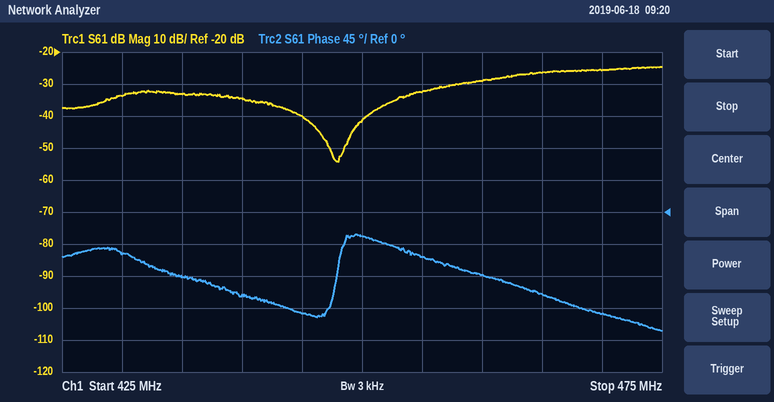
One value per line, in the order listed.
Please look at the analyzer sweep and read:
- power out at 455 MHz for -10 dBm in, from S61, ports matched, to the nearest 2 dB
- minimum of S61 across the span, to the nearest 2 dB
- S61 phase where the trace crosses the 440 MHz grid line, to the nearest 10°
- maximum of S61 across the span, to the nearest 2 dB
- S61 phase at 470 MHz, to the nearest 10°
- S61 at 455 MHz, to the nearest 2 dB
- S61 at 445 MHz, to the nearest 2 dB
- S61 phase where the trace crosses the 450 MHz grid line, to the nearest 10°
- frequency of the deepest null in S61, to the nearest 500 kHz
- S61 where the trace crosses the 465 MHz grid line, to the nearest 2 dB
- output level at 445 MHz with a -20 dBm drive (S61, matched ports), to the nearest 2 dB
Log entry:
-42 dBm
-54 dB
-120°
-24 dB
-140°
-32 dB
-40 dB
-30°
448.0 MHz
-26 dB
-60 dBm
